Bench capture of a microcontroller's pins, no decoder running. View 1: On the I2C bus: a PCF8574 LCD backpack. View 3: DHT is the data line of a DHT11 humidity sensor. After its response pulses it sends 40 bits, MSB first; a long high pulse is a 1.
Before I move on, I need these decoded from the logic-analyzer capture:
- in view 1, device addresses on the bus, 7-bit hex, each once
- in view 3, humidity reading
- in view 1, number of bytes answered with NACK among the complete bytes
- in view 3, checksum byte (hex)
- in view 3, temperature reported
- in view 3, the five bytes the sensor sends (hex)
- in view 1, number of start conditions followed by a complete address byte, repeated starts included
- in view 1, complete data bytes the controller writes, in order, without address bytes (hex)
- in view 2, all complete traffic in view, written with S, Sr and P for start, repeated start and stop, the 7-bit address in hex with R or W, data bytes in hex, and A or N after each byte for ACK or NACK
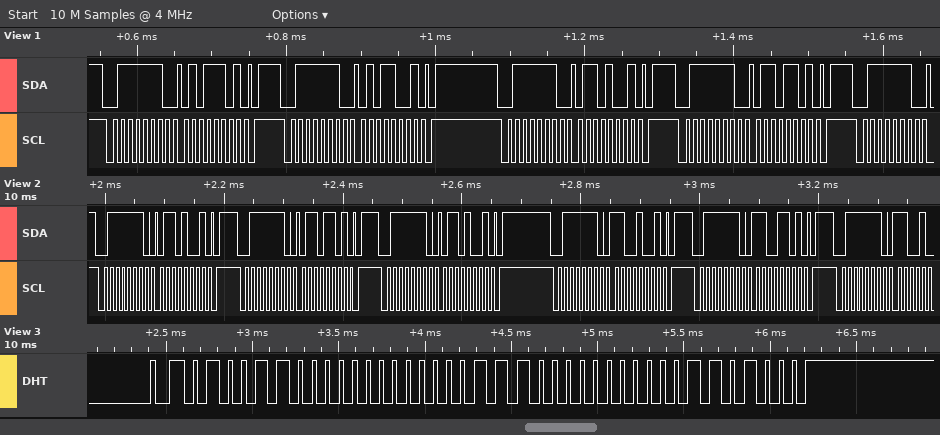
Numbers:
0x3F
76 %
0
0x68
28.0 °C
4C 00 1C 00 68
5
5D 59 69 6D
S 3FW A 69 A P S 3FW A 6D A P S 3FW A 69 A P S 3FW A C9 A P S 3FW A CD A P S 3FW A
